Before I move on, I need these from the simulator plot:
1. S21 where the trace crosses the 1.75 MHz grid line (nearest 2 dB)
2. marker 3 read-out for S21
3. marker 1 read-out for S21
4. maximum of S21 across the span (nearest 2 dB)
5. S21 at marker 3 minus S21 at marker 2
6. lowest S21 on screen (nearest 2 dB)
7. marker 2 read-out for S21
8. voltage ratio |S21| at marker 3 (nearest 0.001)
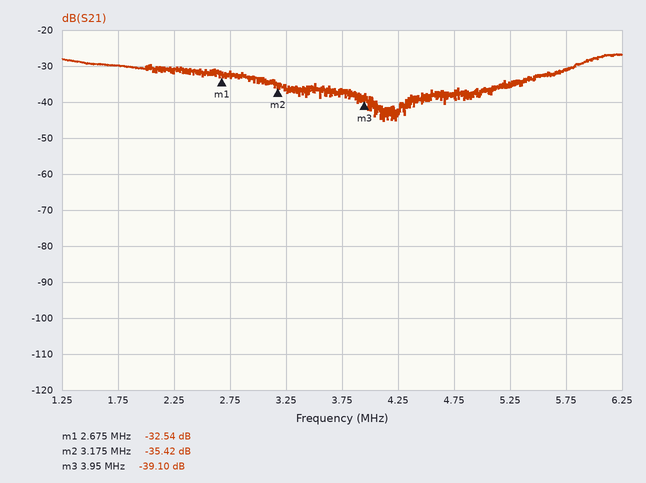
-30 dB
-39.10 dB
-32.54 dB
-26 dB
-3.68 dB
-46 dB
-35.42 dB
0.011
